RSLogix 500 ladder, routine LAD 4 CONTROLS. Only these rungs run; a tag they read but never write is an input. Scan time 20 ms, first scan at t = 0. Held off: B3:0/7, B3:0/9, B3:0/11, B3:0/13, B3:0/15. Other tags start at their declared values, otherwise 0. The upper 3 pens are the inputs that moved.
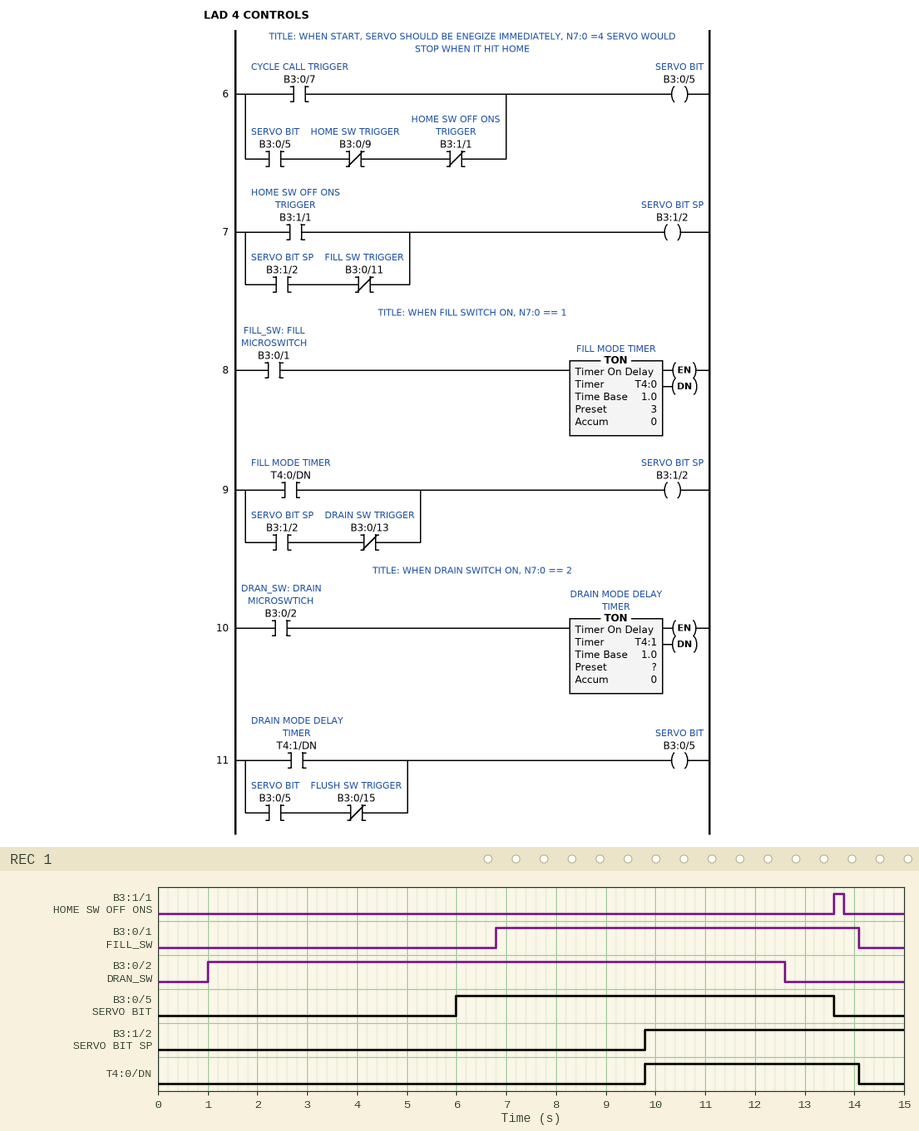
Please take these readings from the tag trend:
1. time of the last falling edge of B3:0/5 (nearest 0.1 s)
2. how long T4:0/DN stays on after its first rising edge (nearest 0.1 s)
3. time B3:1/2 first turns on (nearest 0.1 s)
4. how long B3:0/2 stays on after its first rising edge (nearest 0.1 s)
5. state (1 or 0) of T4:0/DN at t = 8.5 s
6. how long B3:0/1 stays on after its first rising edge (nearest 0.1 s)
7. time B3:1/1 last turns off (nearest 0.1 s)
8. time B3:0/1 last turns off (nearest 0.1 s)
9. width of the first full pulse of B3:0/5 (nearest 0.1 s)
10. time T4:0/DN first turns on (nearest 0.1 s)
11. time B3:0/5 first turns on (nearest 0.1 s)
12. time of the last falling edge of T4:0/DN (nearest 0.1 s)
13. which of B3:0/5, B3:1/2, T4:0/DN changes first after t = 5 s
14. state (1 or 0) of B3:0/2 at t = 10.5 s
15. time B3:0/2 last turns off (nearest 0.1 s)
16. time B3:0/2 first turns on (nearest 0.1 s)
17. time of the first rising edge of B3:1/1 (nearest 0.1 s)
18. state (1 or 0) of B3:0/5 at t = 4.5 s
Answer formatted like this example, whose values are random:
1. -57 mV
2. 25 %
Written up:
1. 13.6 s
2. 4.3 s
3. 9.8 s
4. 11.6 s
5. 0
6. 7.3 s
7. 13.8 s
8. 14.1 s
9. 7.6 s
10. 9.8 s
11. 6.0 s
12. 14.1 s
13. B3:0/5
14. 1
15. 12.6 s
16. 1.0 s
17. 13.6 s
18. 0
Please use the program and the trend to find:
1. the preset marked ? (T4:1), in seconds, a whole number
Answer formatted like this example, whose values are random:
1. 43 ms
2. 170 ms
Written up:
1. 5 s
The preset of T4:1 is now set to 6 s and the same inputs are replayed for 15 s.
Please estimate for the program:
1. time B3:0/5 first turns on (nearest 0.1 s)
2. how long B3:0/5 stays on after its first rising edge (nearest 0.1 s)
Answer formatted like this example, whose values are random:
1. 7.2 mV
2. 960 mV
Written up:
1. 7.0 s
2. 6.6 s
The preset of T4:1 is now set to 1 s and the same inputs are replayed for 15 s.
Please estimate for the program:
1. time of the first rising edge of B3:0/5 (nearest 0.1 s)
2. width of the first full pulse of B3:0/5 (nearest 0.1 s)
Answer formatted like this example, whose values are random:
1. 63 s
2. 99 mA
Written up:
1. 2.0 s
2. 11.6 s
